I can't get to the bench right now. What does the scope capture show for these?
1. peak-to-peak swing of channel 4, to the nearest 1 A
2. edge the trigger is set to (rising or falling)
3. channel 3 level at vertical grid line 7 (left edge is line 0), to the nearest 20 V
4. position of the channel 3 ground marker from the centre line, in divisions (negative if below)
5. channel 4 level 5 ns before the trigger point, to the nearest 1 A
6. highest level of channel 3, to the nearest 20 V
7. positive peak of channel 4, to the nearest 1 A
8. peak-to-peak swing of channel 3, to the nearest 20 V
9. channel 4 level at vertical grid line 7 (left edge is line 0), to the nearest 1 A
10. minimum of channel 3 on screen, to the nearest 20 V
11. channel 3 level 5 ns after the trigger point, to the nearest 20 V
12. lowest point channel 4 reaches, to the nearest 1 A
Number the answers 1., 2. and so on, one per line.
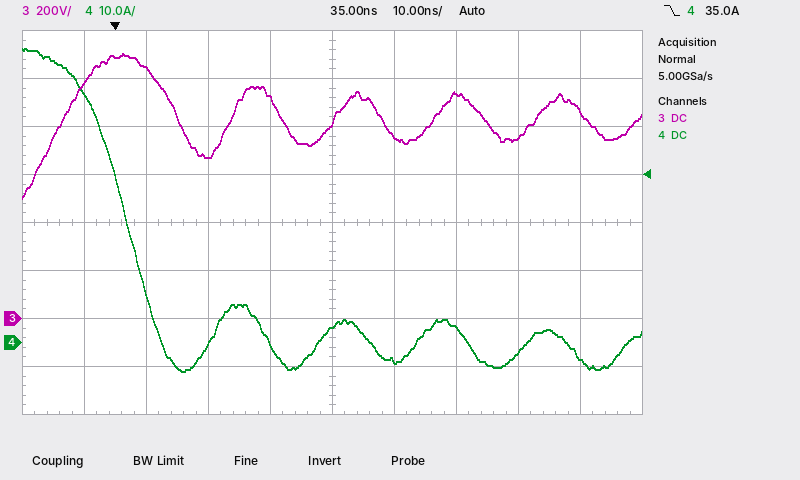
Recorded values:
1. 67 A
2. falling
3. 940 V
4. -2.0 div
5. 52 A
6. 1.10 kV
7. 61 A
8. 600 V
9. 3 A
10. 500 V
11. 1.04 kV
12. -6 A
